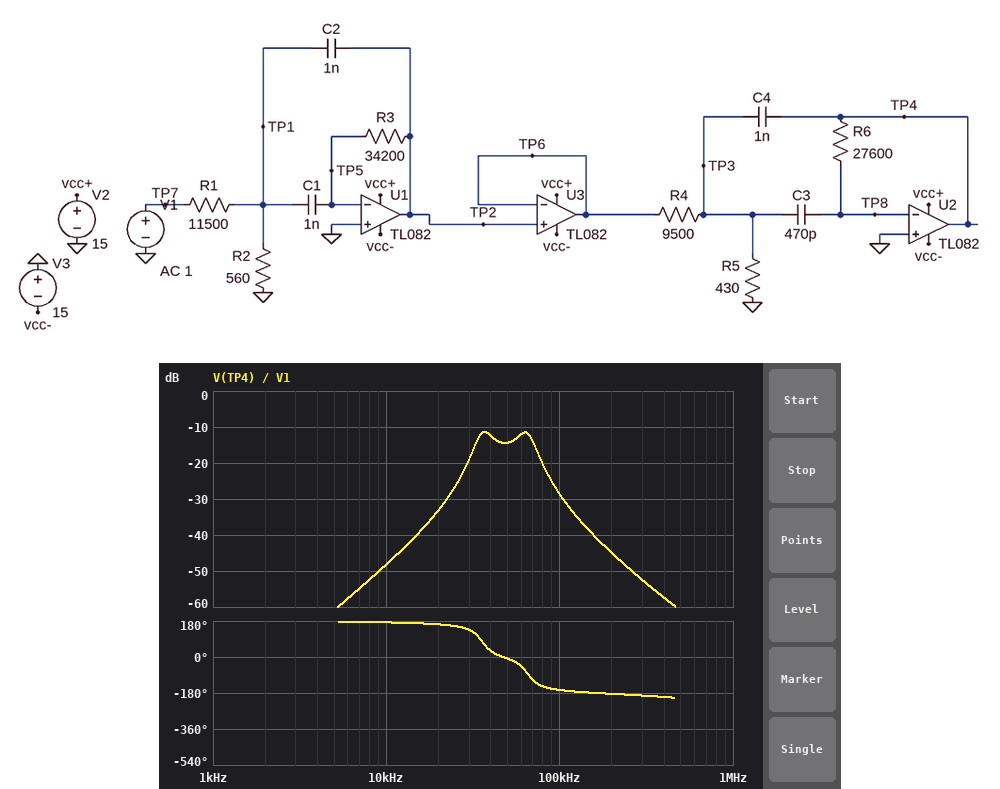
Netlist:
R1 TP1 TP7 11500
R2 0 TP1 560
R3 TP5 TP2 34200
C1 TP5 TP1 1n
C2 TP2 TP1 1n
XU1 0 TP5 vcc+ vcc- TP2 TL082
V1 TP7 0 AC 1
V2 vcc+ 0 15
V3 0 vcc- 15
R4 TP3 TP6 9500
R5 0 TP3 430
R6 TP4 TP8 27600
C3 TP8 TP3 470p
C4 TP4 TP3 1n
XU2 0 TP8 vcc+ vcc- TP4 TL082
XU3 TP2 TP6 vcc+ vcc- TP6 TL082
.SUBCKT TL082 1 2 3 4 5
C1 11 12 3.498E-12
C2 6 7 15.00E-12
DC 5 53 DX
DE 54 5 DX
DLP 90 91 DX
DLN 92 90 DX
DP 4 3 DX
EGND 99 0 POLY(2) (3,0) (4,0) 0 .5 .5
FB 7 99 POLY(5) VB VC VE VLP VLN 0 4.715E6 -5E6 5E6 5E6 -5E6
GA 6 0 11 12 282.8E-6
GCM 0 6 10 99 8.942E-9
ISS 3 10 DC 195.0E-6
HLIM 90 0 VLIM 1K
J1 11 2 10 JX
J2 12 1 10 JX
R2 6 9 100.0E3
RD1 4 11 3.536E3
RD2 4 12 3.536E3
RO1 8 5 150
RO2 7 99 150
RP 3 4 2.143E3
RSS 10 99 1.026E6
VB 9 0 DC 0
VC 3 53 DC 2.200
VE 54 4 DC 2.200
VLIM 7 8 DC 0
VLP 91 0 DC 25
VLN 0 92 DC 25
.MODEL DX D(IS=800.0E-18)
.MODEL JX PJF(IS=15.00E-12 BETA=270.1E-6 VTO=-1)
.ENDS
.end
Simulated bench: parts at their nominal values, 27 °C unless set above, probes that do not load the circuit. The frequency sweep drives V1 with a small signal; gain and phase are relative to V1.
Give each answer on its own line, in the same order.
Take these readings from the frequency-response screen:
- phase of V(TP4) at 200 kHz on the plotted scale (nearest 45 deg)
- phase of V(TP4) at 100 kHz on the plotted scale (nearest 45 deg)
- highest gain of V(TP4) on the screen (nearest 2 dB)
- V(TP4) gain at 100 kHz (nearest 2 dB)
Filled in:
-180 deg
-180 deg
-12 dB
-28 dB
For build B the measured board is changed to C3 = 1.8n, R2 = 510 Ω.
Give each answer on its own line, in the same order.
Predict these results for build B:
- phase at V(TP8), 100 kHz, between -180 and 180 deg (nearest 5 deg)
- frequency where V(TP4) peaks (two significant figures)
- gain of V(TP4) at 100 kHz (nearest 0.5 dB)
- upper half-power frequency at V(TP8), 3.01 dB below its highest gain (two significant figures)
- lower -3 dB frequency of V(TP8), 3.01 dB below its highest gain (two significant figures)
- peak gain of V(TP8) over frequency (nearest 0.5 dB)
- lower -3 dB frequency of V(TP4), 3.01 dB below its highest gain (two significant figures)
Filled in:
100 deg
35 kHz
-32.0 dB
39 kHz
33 kHz
-32.5 dB
32 kHz
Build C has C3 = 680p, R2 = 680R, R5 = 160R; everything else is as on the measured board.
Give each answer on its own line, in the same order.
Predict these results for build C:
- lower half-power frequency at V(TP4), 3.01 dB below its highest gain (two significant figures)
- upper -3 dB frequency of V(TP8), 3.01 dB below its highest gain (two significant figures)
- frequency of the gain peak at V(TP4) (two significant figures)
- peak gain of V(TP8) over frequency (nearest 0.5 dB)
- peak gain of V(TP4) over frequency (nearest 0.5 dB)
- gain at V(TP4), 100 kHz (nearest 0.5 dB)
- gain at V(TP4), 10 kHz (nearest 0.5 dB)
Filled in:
76 kHz
86 kHz
81 kHz
-44.5 dB
-12.0 dB
-25.5 dB
-51.5 dB
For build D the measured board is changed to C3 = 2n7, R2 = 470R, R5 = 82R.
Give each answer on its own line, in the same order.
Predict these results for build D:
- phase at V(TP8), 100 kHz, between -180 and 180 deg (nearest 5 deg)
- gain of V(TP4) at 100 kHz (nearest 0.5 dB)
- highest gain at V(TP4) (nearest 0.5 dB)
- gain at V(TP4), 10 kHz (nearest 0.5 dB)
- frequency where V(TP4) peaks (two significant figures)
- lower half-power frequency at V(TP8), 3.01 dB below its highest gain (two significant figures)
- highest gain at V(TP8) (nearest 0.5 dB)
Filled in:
100 deg
-33.5 dB
2.5 dB
-48.5 dB
51 kHz
49 kHz
-34.0 dB
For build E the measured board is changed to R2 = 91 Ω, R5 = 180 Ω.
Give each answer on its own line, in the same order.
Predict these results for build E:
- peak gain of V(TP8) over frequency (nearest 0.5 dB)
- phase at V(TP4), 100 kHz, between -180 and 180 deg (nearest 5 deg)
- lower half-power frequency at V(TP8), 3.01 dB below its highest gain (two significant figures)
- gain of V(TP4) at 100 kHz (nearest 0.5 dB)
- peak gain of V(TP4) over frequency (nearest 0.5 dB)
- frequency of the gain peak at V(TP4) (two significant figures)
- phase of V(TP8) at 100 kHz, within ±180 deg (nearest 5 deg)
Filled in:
-38.5 dB
-135 deg
72 kHz
-16.5 dB
-5.0 dB
74 kHz
140 deg
